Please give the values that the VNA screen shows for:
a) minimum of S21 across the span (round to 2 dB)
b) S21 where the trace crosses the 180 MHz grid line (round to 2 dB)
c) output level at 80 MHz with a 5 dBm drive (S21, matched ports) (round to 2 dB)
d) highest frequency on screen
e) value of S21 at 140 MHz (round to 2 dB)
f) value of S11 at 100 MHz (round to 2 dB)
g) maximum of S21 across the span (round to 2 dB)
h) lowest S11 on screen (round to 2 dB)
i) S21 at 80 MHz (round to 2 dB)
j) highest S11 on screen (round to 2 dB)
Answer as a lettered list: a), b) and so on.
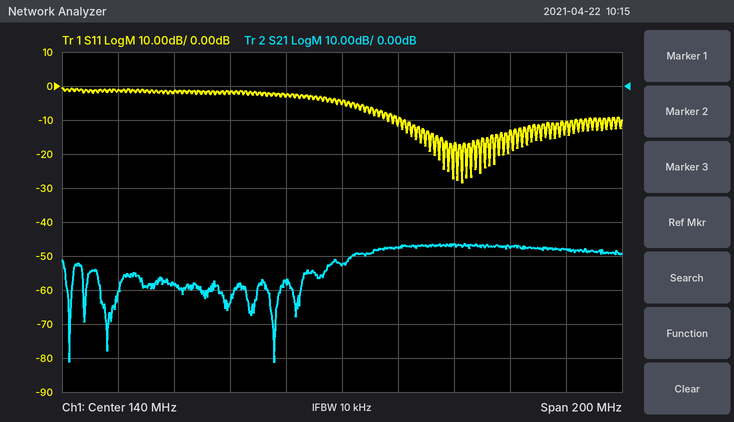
a) -82 dB
b) -46 dB
c) -54 dBm
d) 240 MHz
e) -52 dB
f) -2 dB
g) -46 dB
h) -28 dB
i) -58 dB
j) 0 dB
